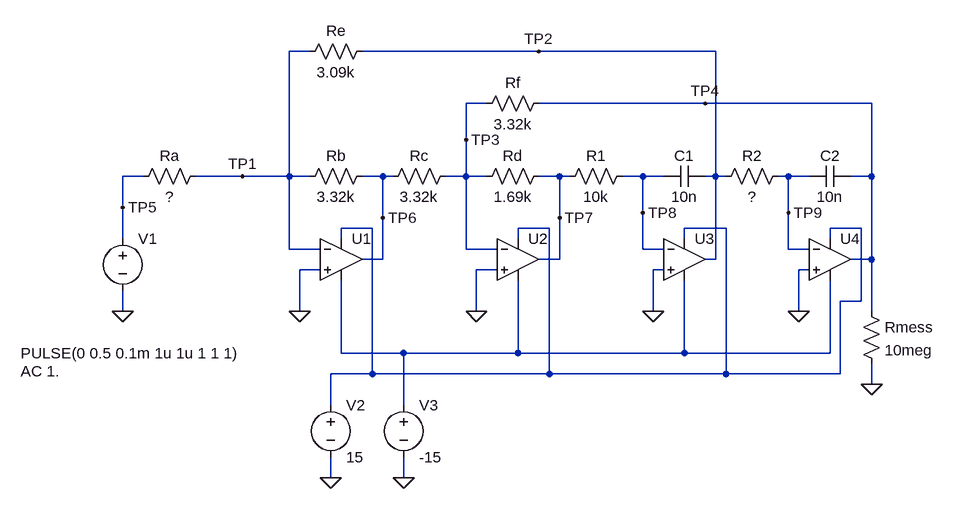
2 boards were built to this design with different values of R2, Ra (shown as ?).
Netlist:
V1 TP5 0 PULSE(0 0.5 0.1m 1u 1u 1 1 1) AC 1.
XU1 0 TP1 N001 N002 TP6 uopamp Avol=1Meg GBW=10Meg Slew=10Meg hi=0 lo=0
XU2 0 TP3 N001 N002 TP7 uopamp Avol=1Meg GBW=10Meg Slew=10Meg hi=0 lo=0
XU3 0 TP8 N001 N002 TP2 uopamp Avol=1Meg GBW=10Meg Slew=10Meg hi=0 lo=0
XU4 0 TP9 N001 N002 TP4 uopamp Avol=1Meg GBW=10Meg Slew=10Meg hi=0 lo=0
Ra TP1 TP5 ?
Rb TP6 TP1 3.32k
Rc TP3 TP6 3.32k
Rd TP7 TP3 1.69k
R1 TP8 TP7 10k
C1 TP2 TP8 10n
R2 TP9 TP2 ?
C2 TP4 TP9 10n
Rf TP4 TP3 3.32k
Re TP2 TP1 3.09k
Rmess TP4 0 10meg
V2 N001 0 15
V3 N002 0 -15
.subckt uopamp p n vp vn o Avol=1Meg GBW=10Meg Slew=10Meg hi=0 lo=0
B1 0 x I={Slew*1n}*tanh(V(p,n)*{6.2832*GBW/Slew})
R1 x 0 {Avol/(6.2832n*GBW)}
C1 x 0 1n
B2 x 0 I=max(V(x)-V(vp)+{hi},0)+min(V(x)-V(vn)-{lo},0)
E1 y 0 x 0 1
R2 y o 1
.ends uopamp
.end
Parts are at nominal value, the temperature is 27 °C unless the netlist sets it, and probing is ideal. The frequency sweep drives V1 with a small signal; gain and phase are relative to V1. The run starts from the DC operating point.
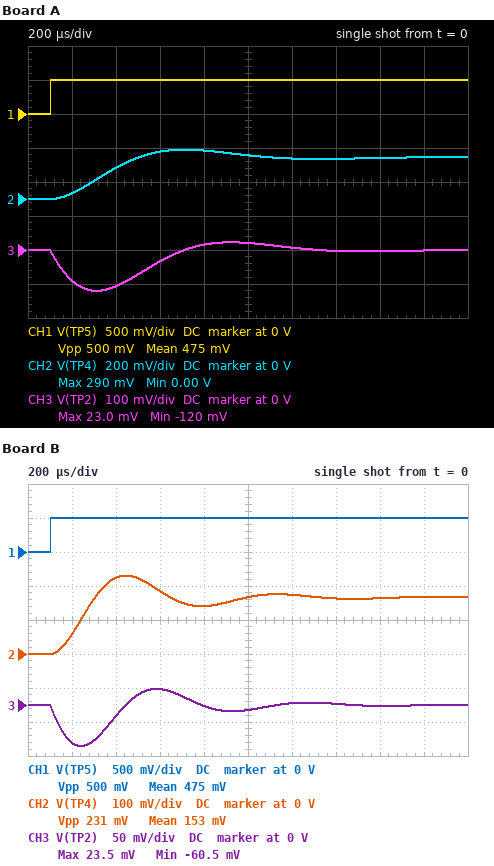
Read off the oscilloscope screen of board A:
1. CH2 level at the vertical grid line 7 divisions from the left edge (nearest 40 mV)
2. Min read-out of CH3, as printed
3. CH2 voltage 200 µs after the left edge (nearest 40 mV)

240 mV
-120 mV
40 mV
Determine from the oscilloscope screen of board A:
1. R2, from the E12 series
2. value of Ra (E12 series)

15 kΩ
6.8 kΩ
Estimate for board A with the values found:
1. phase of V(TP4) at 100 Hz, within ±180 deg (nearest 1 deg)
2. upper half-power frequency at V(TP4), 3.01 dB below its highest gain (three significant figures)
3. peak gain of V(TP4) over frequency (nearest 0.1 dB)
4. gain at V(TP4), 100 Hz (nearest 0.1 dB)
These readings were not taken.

-6 deg
1.09 kHz
-4.6 dB
-6.2 dB
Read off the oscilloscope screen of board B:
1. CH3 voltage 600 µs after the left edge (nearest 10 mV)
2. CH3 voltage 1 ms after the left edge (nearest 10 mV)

20 mV
-10 mV
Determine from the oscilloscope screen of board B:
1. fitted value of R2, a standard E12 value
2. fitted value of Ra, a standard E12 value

5.6 kΩ
10 kΩ
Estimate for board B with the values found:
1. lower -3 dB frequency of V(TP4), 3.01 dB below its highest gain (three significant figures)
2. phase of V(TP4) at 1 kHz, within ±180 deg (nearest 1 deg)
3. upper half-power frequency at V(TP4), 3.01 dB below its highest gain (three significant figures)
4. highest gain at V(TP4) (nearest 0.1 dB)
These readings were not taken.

812 Hz
-34 deg
1.79 kHz
-4.4 dB
